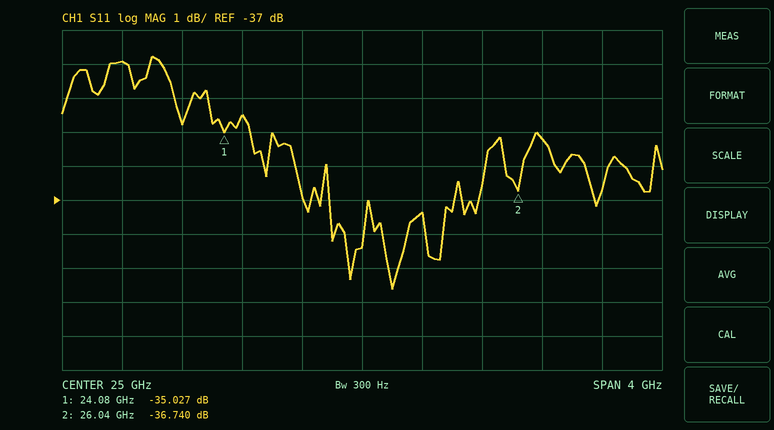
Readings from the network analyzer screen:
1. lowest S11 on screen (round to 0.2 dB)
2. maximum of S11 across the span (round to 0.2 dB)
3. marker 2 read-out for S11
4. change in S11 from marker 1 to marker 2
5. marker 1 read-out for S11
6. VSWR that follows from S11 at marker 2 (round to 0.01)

-39.6 dB
-32.8 dB
-36.740 dB
-1.713 dB
-35.027 dB
1.03
